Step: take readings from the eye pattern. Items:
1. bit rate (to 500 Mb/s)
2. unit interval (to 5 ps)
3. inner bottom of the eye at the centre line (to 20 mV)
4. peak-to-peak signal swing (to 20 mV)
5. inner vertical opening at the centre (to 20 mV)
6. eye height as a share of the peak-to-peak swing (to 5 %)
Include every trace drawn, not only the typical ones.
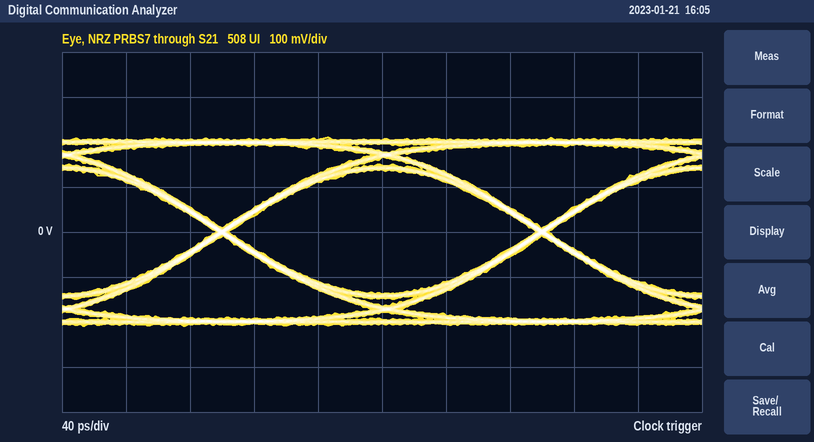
5.0 Gb/s
200 ps
-140 mV
420 mV
280 mV
65 %
